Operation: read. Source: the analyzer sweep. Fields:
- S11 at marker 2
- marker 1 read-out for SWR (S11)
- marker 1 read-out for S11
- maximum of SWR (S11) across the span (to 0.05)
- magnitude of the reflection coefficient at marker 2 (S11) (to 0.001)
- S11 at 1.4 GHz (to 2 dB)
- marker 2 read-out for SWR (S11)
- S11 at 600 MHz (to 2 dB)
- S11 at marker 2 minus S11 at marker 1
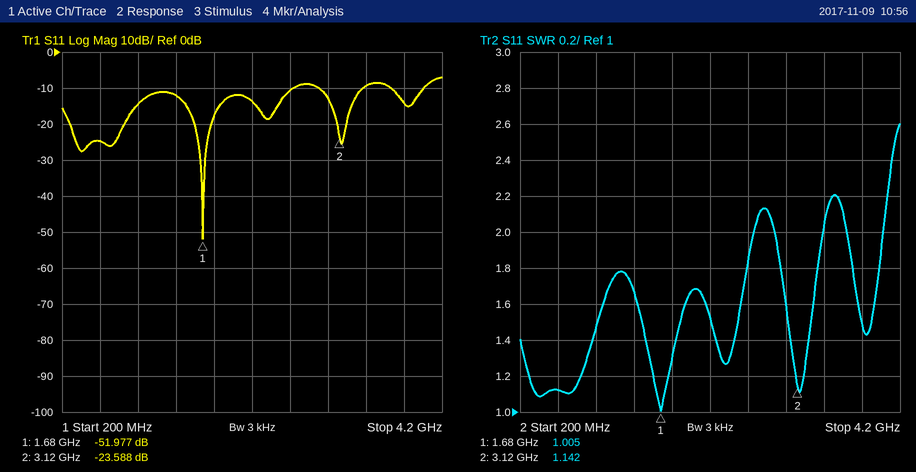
-23.588 dB
1.005
-51.977 dB
2.60
0.066
-12 dB
1.142
-24 dB
28.389 dB
